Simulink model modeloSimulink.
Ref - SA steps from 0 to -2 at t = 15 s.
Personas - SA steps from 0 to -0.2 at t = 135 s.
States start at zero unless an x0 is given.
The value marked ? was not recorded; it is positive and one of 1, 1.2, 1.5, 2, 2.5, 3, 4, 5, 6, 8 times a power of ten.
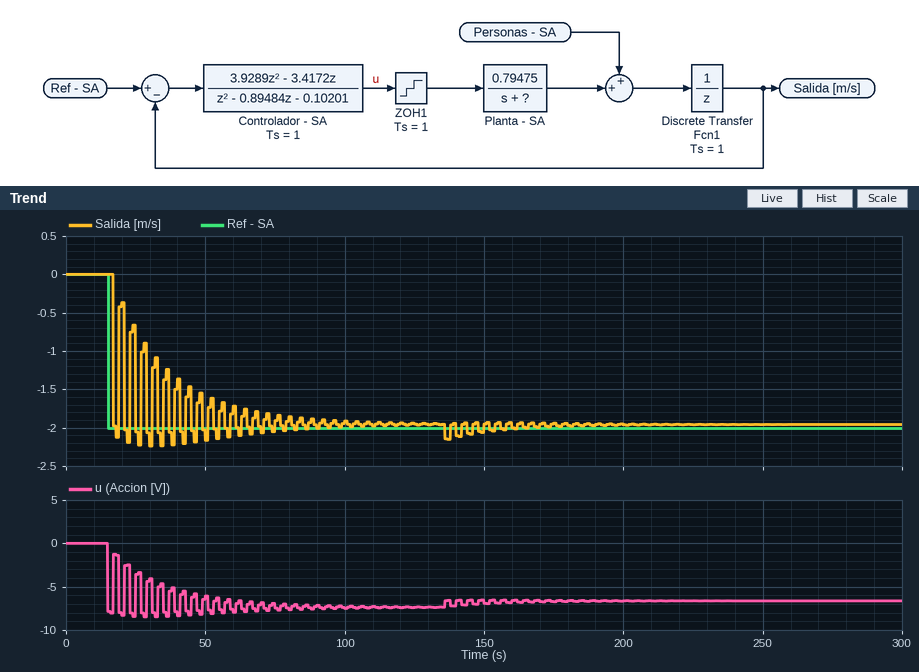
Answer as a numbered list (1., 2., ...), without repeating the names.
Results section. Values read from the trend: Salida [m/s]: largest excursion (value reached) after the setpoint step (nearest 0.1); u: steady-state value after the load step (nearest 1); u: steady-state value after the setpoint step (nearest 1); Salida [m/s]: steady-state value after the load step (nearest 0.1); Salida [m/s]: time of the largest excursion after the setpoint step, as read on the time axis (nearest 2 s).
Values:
1. -2.2
2. -7
3. -7
4. -2.0
5. 30 s
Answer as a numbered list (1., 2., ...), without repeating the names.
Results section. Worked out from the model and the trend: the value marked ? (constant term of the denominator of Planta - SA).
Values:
1. 3
